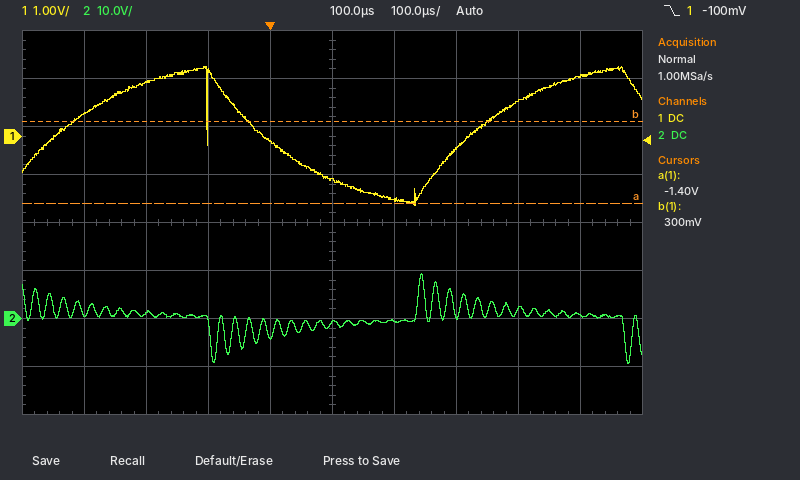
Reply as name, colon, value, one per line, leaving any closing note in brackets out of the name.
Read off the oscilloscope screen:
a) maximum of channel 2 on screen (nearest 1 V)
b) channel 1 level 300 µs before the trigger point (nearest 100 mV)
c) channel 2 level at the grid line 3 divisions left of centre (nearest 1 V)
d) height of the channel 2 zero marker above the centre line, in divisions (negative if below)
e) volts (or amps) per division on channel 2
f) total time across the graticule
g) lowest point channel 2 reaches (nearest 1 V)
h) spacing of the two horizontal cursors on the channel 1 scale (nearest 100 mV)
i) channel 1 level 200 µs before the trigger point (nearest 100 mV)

maximum of channel 2 on screen: 9 V
channel 1 level 300 µs before the trigger point: 500 mV
channel 2 level at the grid line 3 divisions left of centre: 1 V
height of the channel 2 zero marker above the centre line, in divisions: -2.0 div
volts (or amps) per division on channel 2: 10 V
total time across the graticule: 1 ms
lowest point channel 2 reaches: -9 V
spacing of the two horizontal cursors on the channel 1 scale: 1.7 V
channel 1 level 200 µs before the trigger point: 1.1 V
